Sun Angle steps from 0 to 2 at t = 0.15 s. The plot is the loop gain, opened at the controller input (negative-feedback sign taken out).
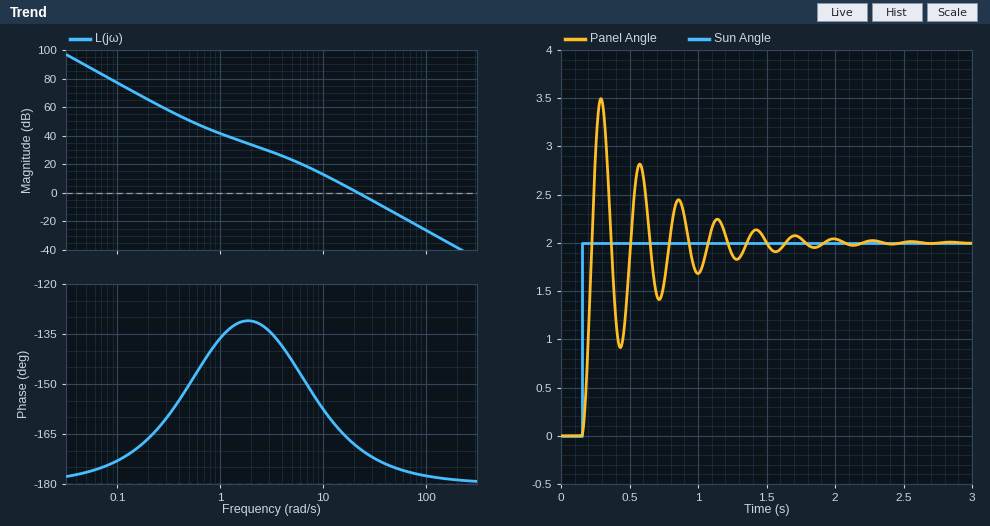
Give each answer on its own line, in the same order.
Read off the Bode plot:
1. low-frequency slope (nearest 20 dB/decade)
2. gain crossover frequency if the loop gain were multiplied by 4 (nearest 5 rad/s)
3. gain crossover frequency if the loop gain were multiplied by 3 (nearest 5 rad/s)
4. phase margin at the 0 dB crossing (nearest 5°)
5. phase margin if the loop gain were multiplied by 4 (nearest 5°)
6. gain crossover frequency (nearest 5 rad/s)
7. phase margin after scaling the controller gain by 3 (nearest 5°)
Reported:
-40 dB/decade
45 rad/s
40 rad/s
10°
5°
20 rad/s
5°
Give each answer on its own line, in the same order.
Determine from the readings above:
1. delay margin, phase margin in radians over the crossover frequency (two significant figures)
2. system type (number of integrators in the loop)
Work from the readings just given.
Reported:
0.0087 s
2
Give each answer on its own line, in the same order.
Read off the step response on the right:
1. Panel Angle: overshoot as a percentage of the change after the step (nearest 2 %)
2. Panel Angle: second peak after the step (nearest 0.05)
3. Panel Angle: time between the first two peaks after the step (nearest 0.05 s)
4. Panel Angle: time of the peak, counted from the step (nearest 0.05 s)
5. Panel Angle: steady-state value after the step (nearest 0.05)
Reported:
74 %
2.80
0.30 s
0.15 s
2.00
